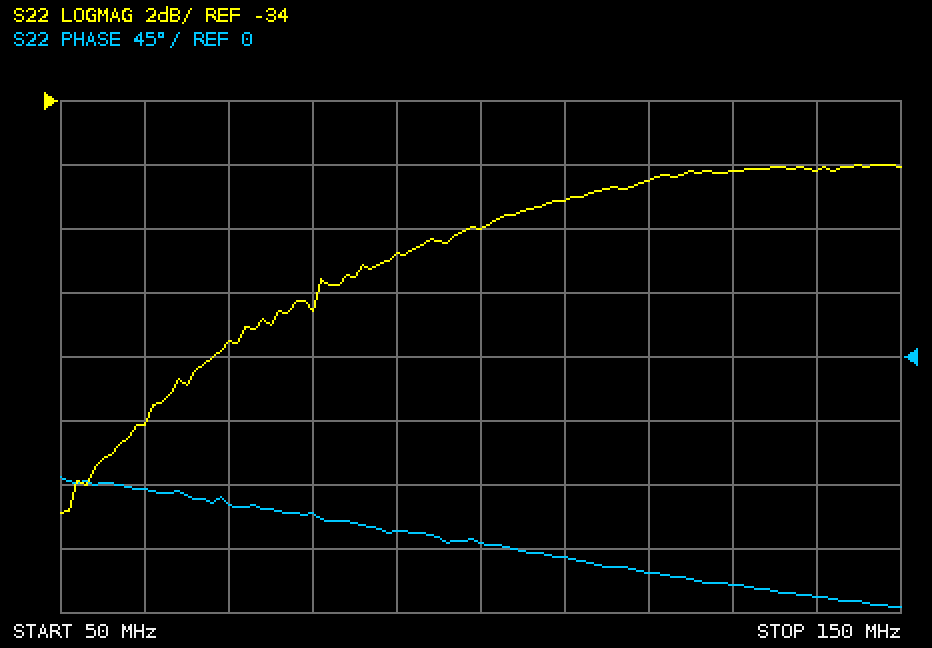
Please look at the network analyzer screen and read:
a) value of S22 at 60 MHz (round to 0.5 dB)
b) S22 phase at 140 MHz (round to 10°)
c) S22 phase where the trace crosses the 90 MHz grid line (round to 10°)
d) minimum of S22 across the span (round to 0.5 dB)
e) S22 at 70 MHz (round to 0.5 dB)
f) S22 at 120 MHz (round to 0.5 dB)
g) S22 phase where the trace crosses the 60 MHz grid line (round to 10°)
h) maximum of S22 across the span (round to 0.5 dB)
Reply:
-44.0 dB
-170°
-120°
-47.0 dB
-41.5 dB
-36.5 dB
-90°
-36.0 dB
